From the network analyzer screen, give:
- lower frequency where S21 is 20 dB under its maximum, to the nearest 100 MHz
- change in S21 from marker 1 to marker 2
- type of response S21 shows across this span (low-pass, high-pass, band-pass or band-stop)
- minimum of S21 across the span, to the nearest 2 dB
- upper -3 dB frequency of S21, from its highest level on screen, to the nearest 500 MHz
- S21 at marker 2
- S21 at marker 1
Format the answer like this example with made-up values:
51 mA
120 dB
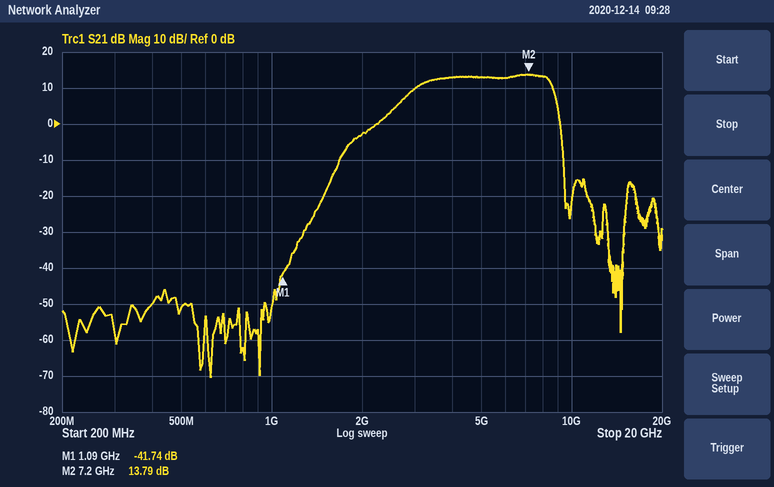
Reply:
1.8 GHz
55.53 dB
band-pass
-70 dB
8.5 GHz
13.79 dB
-41.74 dB
